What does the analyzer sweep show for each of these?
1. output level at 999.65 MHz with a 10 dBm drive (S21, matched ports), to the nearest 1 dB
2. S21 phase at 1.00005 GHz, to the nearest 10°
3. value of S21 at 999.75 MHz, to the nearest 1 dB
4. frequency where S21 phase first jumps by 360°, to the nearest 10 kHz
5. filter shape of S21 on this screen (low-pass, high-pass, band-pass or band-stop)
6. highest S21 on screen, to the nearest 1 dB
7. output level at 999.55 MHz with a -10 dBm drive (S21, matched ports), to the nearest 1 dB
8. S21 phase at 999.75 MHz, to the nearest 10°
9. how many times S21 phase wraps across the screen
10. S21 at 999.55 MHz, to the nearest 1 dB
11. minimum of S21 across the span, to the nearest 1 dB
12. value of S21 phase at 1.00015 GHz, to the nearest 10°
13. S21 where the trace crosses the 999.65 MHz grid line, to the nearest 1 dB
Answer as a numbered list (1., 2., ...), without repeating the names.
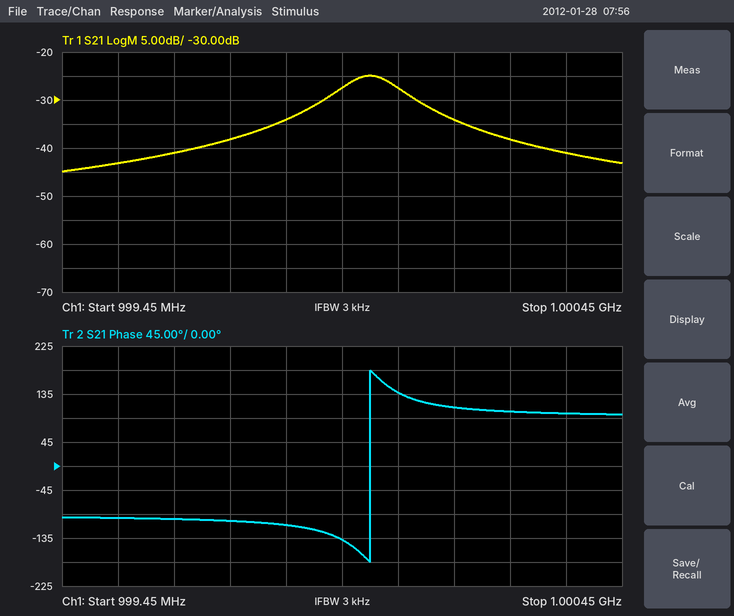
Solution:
1. -31 dBm
2. 140°
3. -38 dB
4. 1.00000 GHz
5. band-pass
6. -25 dB
7. -53 dBm
8. -100°
9. 1
10. -43 dB
11. -45 dB
12. 110°
13. -41 dB
